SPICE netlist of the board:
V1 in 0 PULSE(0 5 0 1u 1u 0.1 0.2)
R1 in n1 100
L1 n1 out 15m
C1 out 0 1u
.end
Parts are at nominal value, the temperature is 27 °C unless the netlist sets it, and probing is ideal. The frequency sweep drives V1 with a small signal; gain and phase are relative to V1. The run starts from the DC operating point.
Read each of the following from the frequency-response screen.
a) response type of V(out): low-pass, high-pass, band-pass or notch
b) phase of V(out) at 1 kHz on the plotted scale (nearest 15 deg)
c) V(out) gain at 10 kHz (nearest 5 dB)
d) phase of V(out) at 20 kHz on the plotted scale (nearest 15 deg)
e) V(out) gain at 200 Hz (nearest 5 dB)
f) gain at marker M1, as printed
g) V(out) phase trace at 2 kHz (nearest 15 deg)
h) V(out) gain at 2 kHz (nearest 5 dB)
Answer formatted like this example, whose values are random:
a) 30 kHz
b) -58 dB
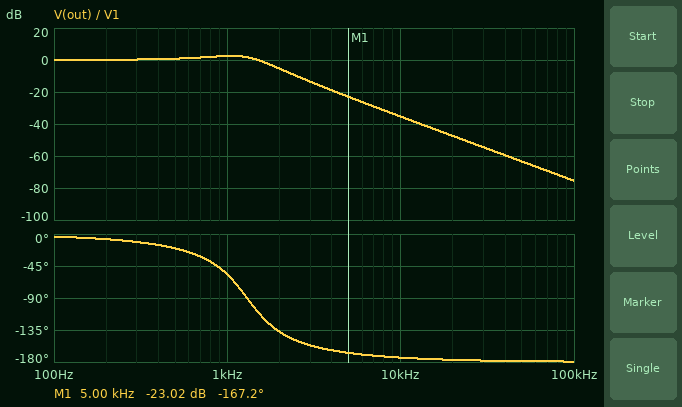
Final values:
a) low-pass
b) -60 deg
c) -35 dB
d) -180 deg
e) 0 dB
f) -23.02 dB
g) -135 deg
h) -5 dB
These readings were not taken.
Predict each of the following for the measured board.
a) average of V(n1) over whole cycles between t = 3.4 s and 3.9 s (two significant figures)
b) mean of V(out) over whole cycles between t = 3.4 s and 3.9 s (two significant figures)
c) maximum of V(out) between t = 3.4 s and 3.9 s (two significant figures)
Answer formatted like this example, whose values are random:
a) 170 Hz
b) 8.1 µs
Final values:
a) 2.5 V
b) 2.5 V
c) 6.3 V
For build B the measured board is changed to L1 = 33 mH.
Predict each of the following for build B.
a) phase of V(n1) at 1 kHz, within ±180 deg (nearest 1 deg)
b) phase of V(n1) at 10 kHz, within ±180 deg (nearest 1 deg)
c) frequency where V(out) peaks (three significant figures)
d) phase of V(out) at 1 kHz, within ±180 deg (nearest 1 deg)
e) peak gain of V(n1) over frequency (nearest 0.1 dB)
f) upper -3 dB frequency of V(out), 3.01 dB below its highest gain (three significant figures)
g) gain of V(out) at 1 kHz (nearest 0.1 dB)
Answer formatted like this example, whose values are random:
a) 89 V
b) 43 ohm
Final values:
a) 64 deg
b) 3 deg
c) 807 Hz
d) -116 deg
e) 0 dB
f) 1.03 kHz
g) 3.1 dB
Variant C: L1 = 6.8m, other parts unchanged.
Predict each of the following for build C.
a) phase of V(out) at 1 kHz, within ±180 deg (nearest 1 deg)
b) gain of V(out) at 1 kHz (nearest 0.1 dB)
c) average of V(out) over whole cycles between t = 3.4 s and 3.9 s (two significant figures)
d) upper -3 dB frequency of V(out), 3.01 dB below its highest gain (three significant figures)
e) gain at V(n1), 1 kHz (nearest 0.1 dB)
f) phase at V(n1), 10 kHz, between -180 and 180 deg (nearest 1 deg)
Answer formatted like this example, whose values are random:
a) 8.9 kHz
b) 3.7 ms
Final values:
a) -41 deg
b) 0.3 dB
c) 2.5 V
d) 2.14 kHz
e) -2.4 dB
f) 14 deg
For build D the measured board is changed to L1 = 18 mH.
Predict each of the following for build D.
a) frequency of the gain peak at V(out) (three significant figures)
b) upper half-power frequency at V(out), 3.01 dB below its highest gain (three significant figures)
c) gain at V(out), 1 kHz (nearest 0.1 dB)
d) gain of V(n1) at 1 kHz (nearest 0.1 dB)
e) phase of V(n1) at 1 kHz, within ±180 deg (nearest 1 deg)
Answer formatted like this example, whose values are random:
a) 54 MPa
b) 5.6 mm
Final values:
a) 1.01 kHz
b) 1.41 kHz
c) 3.2 dB
d) -7.6 dB
e) -65 deg
